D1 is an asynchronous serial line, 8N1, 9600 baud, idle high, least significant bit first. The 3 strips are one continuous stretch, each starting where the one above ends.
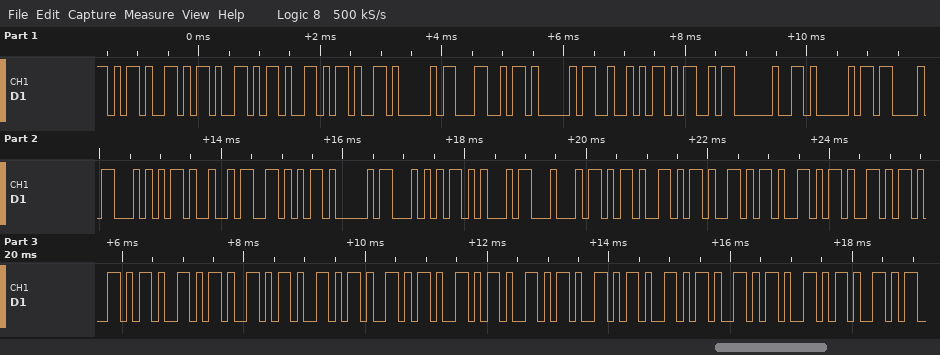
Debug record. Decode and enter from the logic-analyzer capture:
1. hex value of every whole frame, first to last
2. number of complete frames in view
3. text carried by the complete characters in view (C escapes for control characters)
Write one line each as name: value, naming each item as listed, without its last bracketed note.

hex value of every whole frame, first to last: 2D 2D 2D 2D 41 4C 41 52 4D 20 41 43 54 49 56 41 54 45 44 2D 2D 2D 2D 2D 2D 2D 2D 2D 2D 2D 2D 2D 2D 2D 2D
number of complete frames in view: 35
text carried by the complete characters in view: "----ALARM ACTIVATED----------------"
